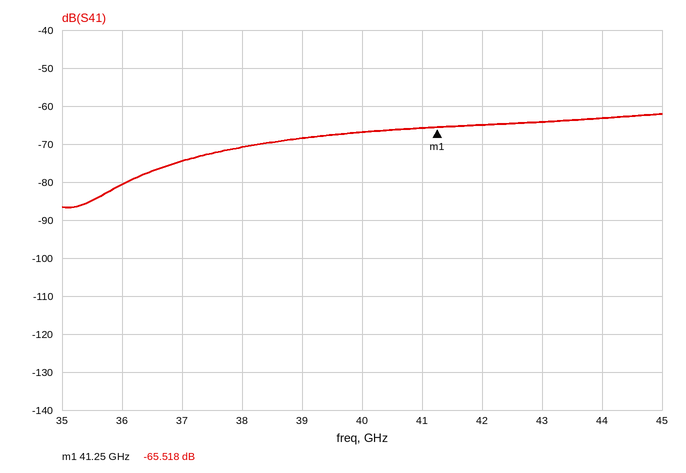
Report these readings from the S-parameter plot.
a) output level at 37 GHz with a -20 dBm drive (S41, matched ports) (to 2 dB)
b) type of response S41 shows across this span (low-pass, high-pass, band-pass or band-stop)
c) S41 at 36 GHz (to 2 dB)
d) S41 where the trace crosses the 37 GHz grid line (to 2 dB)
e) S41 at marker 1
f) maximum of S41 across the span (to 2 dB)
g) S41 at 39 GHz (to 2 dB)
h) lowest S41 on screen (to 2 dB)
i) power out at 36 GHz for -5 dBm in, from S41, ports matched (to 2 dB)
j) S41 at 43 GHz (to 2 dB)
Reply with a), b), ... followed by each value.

a) -94 dBm
b) high-pass
c) -80 dB
d) -74 dB
e) -65.518 dB
f) -62 dB
g) -68 dB
h) -86 dB
i) -86 dBm
j) -64 dB
